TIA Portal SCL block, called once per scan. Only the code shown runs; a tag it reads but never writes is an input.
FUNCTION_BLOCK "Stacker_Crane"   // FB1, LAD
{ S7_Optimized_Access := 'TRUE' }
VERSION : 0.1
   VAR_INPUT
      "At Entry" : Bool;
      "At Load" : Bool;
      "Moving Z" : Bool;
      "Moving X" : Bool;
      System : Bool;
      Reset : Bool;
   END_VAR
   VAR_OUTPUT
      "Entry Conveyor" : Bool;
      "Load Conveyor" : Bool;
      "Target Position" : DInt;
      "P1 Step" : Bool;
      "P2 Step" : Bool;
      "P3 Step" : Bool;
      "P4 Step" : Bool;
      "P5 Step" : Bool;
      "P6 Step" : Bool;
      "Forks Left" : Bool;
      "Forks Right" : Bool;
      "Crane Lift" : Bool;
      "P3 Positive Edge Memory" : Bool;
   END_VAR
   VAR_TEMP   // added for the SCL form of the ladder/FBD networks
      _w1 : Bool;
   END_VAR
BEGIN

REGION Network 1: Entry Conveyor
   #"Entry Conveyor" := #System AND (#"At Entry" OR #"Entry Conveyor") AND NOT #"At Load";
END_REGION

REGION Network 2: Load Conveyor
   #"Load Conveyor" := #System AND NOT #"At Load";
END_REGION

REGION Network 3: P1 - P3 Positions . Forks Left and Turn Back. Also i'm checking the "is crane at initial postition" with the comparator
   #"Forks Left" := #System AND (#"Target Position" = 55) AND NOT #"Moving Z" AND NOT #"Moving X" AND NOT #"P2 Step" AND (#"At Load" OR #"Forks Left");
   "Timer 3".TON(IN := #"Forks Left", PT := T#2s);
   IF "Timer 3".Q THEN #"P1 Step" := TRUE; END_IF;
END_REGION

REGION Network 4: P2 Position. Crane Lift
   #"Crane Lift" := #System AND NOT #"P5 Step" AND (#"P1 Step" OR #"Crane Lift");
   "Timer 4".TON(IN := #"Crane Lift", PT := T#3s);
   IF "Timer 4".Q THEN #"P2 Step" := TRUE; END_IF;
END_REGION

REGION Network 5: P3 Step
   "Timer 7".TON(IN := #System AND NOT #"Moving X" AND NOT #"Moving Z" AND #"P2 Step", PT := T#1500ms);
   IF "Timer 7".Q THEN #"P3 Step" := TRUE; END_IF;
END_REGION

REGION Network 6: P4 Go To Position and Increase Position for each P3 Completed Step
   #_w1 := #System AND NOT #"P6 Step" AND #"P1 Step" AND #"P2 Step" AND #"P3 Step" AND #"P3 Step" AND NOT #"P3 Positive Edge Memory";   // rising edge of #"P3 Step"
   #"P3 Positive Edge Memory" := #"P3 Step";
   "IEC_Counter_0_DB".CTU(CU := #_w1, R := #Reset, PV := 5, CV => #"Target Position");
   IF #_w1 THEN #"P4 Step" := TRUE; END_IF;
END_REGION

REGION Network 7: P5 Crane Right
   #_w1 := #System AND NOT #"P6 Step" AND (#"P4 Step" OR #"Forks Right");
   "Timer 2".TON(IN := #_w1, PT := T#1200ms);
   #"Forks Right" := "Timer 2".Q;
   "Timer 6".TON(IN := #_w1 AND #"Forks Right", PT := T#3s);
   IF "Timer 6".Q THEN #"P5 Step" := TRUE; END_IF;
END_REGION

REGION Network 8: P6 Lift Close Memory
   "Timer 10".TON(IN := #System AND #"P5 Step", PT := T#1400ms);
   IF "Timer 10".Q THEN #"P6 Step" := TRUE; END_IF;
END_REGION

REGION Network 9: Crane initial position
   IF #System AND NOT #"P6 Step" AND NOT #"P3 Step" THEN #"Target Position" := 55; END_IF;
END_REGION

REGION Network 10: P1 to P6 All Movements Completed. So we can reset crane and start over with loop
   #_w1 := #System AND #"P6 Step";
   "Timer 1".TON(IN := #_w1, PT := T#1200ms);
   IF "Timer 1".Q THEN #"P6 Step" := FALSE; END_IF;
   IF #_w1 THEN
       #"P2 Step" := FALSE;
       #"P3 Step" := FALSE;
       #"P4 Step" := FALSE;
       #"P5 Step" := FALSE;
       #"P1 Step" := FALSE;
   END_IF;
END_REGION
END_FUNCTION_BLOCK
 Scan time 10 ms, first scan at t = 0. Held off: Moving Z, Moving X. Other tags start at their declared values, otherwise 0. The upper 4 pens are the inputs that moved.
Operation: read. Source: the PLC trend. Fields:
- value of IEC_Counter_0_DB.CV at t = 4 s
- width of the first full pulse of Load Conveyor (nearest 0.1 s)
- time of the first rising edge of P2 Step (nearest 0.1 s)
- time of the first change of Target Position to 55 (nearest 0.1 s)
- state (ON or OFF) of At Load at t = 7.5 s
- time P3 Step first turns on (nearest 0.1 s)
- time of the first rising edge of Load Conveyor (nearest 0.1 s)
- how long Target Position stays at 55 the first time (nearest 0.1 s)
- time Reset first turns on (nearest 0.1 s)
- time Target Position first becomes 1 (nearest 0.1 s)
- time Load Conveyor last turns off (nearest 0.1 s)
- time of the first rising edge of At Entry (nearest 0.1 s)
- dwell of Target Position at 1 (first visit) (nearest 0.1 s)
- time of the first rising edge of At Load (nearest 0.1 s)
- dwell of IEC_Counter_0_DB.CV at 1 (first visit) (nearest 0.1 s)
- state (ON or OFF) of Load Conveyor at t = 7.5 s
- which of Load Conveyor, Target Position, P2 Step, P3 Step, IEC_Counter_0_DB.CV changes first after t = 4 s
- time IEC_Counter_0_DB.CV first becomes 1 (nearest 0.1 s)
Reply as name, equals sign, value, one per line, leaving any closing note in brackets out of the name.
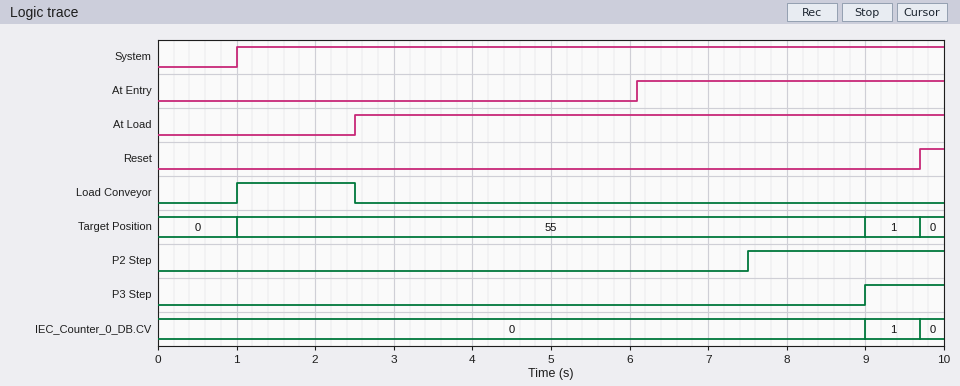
value of IEC_Counter_0_DB.CV at t = 4 s = 0
width of the first full pulse of Load Conveyor = 1.5 s
time of the first rising edge of P2 Step = 7.5 s
time of the first change of Target Position to 55 = 1.0 s
state (ON or OFF) of At Load at t = 7.5 s = ON
time P3 Step first turns on = 9.0 s
time of the first rising edge of Load Conveyor = 1.0 s
how long Target Position stays at 55 the first time = 8.0 s
time Reset first turns on = 9.7 s
time Target Position first becomes 1 = 9.0 s
time Load Conveyor last turns off = 2.5 s
time of the first rising edge of At Entry = 6.1 s
dwell of Target Position at 1 (first visit) = 0.7 s
time of the first rising edge of At Load = 2.5 s
dwell of IEC_Counter_0_DB.CV at 1 (first visit) = 0.7 s
state (ON or OFF) of Load Conveyor at t = 7.5 s = OFF
which of Load Conveyor, Target Position, P2 Step, P3 Step, IEC_Counter_0_DB.CV changes first after t = 4 s = P2 Step
time IEC_Counter_0_DB.CV first becomes 1 = 9.0 s
